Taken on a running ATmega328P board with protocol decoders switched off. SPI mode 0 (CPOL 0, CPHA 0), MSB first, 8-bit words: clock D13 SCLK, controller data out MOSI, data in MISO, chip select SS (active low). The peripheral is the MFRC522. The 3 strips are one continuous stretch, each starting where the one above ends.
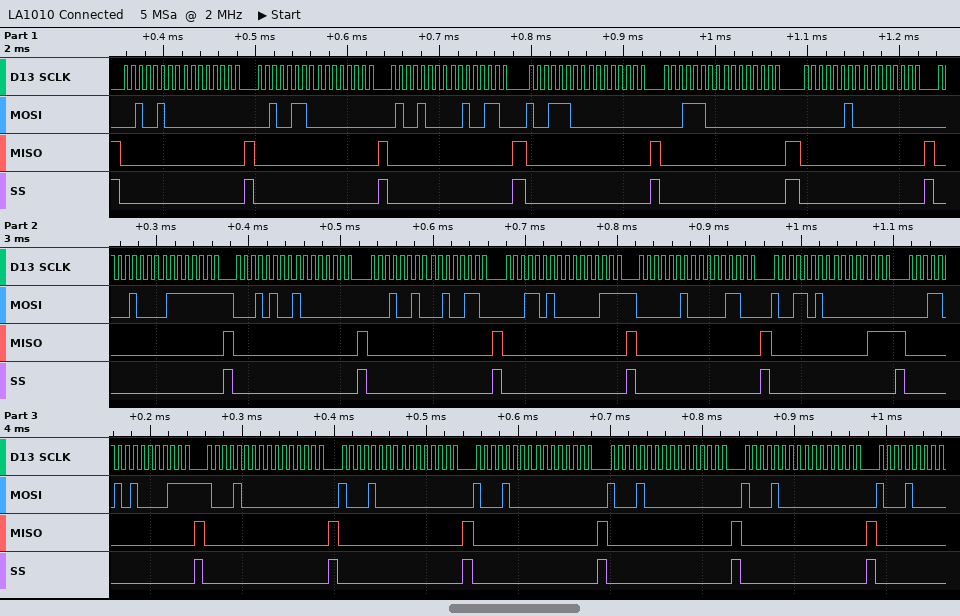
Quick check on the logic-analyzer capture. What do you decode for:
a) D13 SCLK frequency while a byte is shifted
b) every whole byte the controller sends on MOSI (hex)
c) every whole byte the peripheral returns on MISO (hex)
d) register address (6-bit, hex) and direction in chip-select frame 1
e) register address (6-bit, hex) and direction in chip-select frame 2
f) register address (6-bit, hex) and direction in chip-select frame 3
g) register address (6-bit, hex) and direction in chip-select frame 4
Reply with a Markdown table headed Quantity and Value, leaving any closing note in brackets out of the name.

| Quantity | Value |
|---|---|
| D13 SCLK frequency while a byte is shifted | 125 kHz |
| every whole byte the controller sends on MOSI | 24 00 26 00 48 26 9C 00 1C 00 02 00 08 7F 14 80 12 26 1A 07 02 0C 9A 00 1A 87 88 00 88 00 88 00 88 00 88 00 88 |
| every whole byte the peripheral returns on MISO | 00 00 00 00 00 00 00 00 00 00 00 00 00 00 00 00 00 00 00 00 00 00 00 07 00 00 00 00 00 00 00 00 00 00 00 00 00 |
| register address (6-bit, hex) and direction in chip-select frame 1 | 0x12 write |
| register address (6-bit, hex) and direction in chip-select frame 2 | 0x13 write |
| register address (6-bit, hex) and direction in chip-select frame 3 | 0x24 write |
| register address (6-bit, hex) and direction in chip-select frame 4 | 0x0E read |
